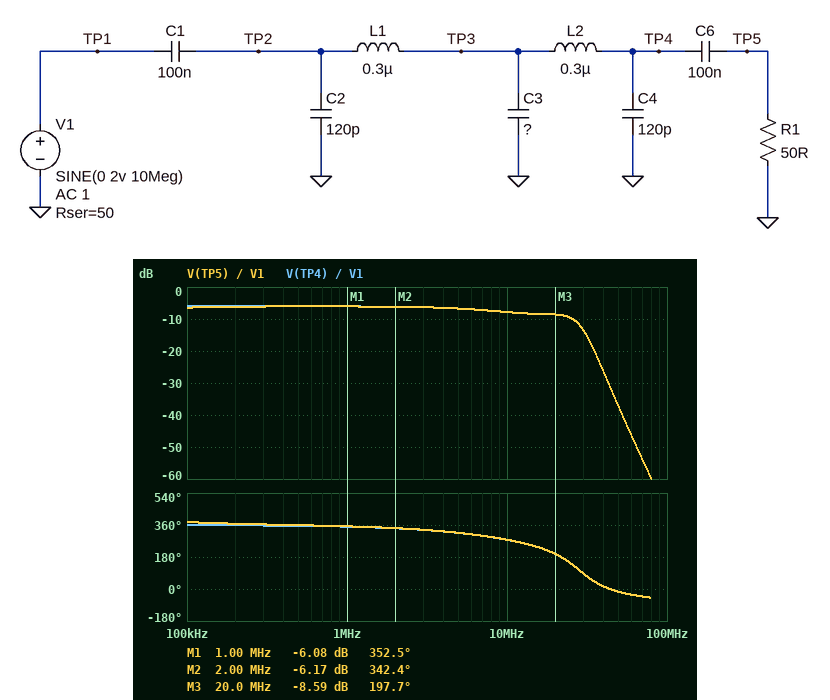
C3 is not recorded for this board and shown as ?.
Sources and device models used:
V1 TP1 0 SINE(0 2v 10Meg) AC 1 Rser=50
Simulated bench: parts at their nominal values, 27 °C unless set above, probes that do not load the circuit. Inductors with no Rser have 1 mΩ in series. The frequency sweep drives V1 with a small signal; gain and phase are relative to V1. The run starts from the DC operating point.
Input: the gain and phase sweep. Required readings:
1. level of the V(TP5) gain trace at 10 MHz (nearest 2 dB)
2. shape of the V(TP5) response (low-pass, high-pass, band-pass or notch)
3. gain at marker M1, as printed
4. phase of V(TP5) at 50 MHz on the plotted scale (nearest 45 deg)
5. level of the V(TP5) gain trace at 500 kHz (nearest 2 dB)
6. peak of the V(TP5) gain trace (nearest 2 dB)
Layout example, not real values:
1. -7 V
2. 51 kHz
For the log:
1. -8 dB
2. low-pass
3. -6.08 dB
4. 0 deg
5. -6 dB
6. -6 dB
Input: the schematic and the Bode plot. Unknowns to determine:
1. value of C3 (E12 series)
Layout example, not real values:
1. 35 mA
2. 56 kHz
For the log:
1. 560 pF
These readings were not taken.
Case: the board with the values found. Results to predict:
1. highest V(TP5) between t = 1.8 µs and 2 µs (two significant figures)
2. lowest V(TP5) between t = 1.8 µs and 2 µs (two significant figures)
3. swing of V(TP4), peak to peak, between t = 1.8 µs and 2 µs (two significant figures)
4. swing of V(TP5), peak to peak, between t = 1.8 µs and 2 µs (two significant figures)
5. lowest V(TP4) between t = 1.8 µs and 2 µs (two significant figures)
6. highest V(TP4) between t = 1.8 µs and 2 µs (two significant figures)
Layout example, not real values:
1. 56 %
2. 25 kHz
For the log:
1. 810 mV
2. -810 mV
3. 1.6 V
4. 1.6 V
5. -810 mV
6. 810 mV
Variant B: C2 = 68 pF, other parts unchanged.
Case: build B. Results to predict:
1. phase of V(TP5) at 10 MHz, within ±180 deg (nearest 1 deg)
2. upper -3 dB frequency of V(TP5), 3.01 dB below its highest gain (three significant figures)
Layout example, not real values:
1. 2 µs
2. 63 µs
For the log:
1. -81 deg
2. 17.3 MHz
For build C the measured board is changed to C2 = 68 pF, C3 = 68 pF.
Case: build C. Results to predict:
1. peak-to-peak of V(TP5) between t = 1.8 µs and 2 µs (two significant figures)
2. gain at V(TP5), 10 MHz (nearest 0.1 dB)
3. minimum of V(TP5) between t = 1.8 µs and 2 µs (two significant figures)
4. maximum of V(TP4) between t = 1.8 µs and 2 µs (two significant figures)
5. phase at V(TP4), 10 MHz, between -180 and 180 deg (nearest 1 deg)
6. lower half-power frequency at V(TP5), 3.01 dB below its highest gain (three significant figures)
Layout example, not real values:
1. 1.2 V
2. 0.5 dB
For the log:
1. 2.0 V
2. -6.0 dB
3. -1.0 V
4. 1.0 V
5. -45 deg
6. 31.9 kHz
